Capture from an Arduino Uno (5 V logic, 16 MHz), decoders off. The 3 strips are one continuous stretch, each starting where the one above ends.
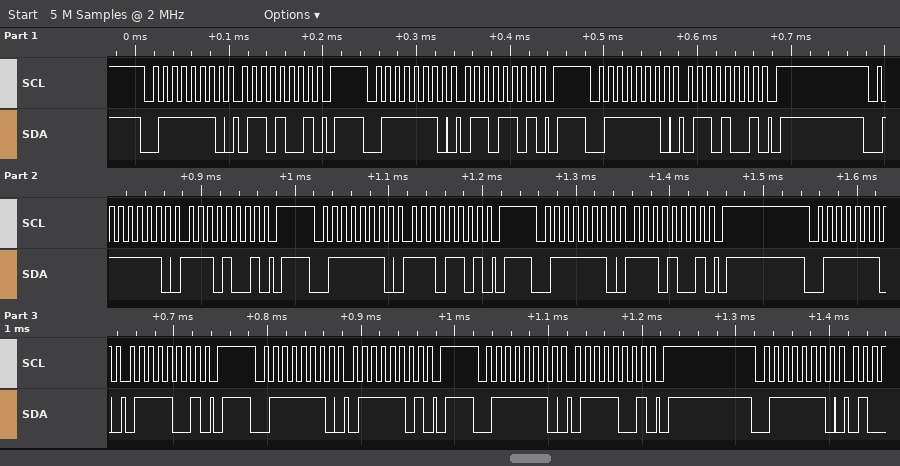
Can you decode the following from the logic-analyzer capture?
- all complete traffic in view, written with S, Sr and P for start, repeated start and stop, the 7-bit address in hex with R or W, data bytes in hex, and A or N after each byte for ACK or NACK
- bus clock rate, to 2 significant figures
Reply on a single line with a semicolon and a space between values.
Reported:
S 3FW A 69 A P S 3FW A 6D A P S 3FW A 69 A P S 3FW A E9 A P S 3FW A ED A P S 3FW A E9 A P S 3FW A 79 A P S 3FW A 7D A P S 3FW A 79 A P S 3FW A; 100 kHz
